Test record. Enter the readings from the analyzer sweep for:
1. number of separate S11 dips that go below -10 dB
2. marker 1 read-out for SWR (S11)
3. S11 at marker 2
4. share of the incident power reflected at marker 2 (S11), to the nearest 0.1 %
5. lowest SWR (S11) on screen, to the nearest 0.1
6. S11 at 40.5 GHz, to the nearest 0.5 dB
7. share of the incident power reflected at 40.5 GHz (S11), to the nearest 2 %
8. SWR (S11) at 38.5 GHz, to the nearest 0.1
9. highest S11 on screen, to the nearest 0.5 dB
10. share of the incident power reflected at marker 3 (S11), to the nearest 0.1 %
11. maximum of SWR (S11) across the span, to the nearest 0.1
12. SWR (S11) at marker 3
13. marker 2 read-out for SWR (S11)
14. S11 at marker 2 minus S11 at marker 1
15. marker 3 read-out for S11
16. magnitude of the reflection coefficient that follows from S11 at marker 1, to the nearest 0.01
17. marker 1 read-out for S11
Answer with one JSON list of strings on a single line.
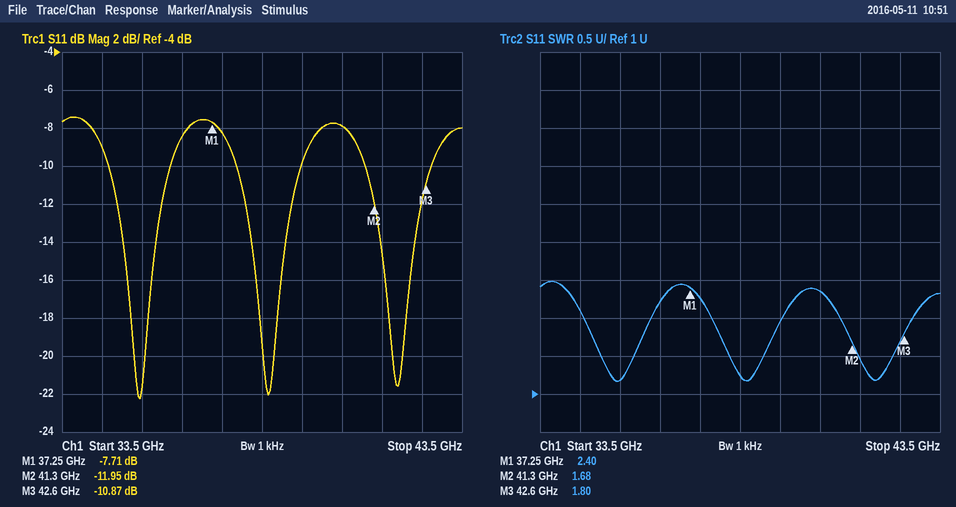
["3", "2.40", "-11.95 dB", "6.4 %", "1.2", "-8.0 dB", "16 %", "1.2", "-7.5 dB", "8.2 %", "2.5", "1.80", "1.68", "-4.24 dB", "-10.87 dB", "0.41", "-7.71 dB"]
